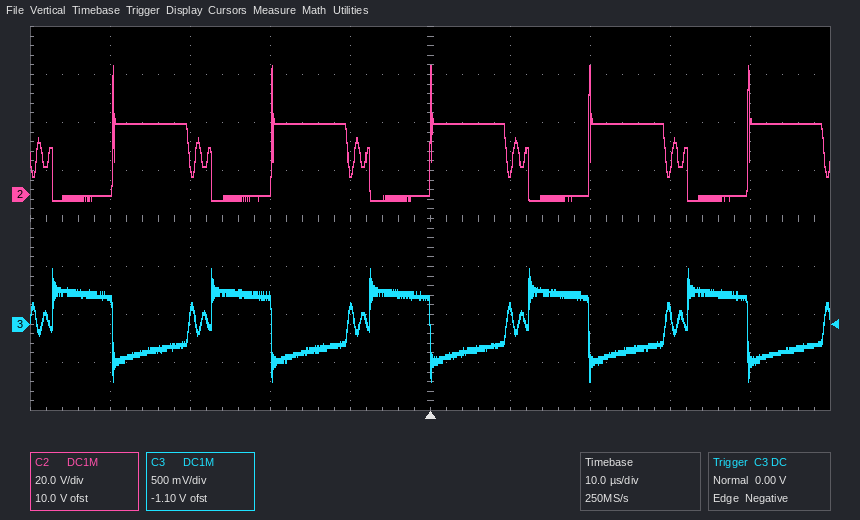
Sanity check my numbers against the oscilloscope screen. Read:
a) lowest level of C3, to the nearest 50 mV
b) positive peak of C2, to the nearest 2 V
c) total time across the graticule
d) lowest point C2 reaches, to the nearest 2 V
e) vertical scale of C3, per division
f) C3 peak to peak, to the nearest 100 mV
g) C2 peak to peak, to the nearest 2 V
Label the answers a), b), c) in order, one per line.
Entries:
a) -600 mV
b) 54 V
c) 100 µs
d) -2 V
e) 500 mV
f) 1.20 V
g) 56 V
